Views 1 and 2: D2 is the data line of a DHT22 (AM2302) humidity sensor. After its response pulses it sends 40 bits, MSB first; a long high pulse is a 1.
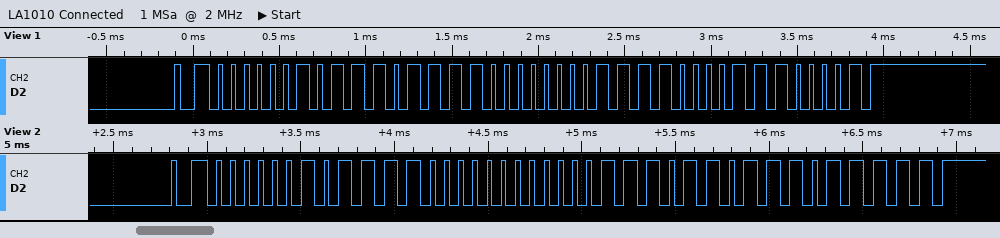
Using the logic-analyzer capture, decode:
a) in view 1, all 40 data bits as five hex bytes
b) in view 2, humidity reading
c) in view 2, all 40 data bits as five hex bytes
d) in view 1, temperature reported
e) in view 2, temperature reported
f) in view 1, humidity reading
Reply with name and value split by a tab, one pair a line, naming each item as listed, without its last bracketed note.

in view 1, all 40 data bits as five hex bytes	02 EF 00 F0 E1
in view 2, humidity reading	75.2 %
in view 2, all 40 data bits as five hex bytes	02 F0 00 ED DF
in view 1, temperature reported	24.0 °C
in view 2, temperature reported	23.7 °C
in view 1, humidity reading	75.1 %
